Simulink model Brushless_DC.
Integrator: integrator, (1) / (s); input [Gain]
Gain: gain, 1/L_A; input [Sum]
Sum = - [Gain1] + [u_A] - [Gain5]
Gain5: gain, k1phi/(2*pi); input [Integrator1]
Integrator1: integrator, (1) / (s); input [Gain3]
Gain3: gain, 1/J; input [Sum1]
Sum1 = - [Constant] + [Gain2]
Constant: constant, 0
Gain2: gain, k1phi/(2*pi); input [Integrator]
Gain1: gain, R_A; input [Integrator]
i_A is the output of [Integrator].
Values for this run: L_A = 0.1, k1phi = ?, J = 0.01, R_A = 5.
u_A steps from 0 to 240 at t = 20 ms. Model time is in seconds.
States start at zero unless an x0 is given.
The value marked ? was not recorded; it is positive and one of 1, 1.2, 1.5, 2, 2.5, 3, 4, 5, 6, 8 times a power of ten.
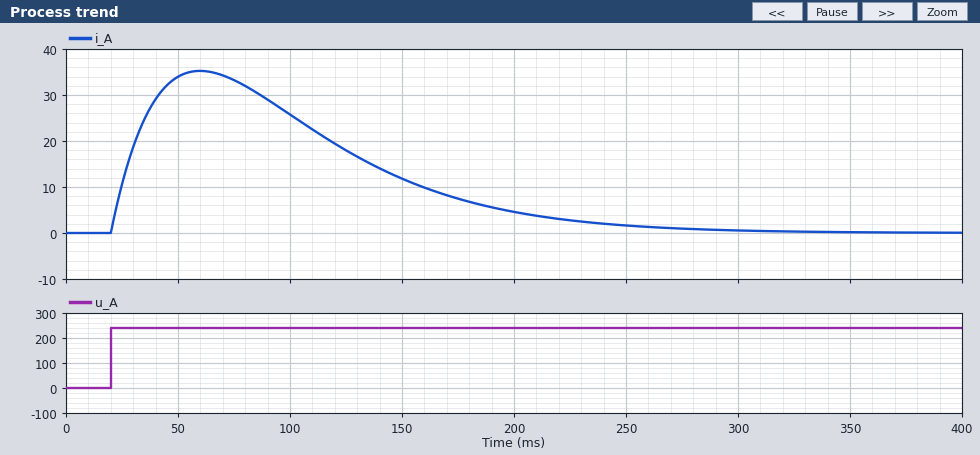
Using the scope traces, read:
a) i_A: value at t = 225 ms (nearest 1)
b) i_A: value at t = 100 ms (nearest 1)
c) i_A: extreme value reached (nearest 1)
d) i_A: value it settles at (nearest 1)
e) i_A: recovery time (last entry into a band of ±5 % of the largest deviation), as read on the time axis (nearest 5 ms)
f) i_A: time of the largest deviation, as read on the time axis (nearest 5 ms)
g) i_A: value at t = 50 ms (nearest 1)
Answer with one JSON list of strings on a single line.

["3", "26", "35", "0", "245 ms", "60 ms", "34"]
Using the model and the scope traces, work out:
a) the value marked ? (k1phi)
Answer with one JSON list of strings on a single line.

["5"]
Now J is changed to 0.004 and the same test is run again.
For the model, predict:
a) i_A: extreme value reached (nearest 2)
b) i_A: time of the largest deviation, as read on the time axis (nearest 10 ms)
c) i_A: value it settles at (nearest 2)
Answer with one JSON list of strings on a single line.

["30", "50 ms", "0"]
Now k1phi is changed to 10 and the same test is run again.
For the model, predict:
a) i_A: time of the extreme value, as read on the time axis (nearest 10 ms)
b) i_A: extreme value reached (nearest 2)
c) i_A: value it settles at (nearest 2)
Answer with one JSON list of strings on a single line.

["40 ms", "26", "0"]
